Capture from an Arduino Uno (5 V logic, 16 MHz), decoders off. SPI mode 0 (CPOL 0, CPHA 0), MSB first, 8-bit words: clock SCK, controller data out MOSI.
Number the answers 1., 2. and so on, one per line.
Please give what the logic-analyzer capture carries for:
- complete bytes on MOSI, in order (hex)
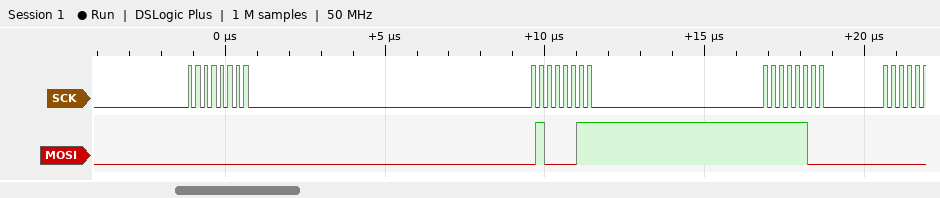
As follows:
1. 0x00 0x43 0xFC
